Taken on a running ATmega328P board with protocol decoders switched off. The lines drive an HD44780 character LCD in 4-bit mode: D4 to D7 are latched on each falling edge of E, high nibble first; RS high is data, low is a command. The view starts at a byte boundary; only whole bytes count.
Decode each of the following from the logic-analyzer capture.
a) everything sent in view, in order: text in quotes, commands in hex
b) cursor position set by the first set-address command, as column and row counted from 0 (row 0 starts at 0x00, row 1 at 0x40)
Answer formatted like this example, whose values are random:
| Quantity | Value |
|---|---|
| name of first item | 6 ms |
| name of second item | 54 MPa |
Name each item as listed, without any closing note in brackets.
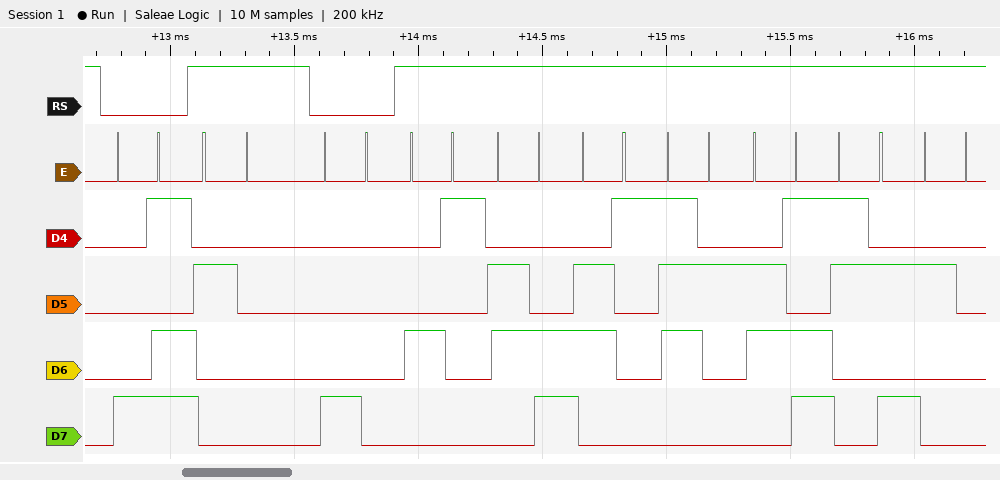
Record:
| Quantity | Value |
|---|---|
| everything sent in view, in order: text in quotes, commands in hex | 0x8D " " 0x80 "Alarm: " |
| cursor position set by the first set-address command, as column and row counted from 0 | column 13, row 0 |
